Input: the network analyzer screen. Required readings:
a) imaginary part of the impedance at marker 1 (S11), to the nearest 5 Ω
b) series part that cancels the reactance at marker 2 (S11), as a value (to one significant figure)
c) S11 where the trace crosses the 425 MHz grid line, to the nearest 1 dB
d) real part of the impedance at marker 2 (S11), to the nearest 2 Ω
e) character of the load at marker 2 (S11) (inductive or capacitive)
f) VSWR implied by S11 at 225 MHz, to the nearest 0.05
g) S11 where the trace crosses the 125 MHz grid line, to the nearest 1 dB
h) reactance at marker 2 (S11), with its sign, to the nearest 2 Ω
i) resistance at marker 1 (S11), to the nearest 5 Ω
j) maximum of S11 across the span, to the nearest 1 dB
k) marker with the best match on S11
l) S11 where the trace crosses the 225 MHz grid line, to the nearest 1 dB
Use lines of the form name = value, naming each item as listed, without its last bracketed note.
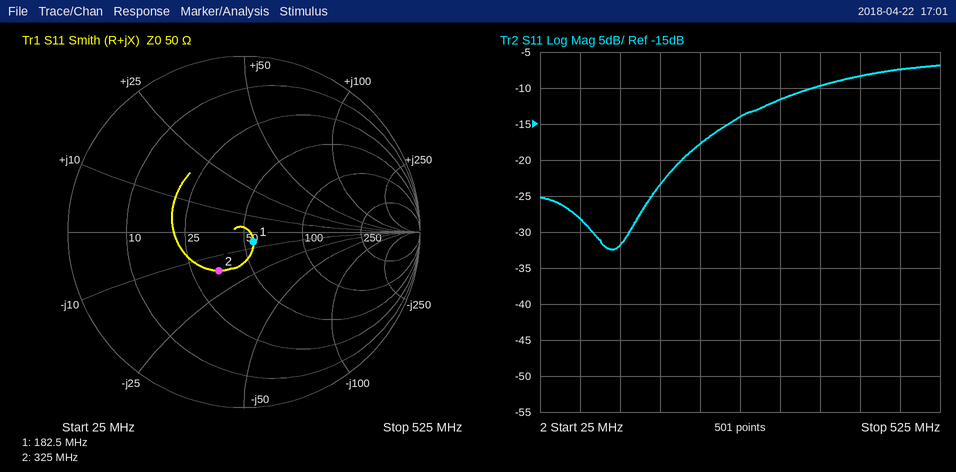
imaginary part of the impedance at marker 1 (S11), to the nearest 5 Ω = -5 Ω
series part that cancels the reactance at marker 2 (S11), as a value = 8 nH
S11 where the trace crosses the 425 MHz grid line, to the nearest 1 dB = -8 dB
real part of the impedance at marker 2 (S11), to the nearest 2 Ω = 34 Ω
character of the load at marker 2 (S11) = capacitive
VSWR implied by S11 at 225 MHz, to the nearest 0.05 = 1.30
S11 where the trace crosses the 125 MHz grid line, to the nearest 1 dB = -32 dB
reactance at marker 2 (S11), with its sign, to the nearest 2 Ω = -16 Ω
resistance at marker 1 (S11), to the nearest 5 Ω = 55 Ω
maximum of S11 across the span, to the nearest 1 dB = -7 dB
marker with the best match on S11 = marker 1
S11 where the trace crosses the 225 MHz grid line, to the nearest 1 dB = -18 dB
